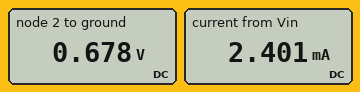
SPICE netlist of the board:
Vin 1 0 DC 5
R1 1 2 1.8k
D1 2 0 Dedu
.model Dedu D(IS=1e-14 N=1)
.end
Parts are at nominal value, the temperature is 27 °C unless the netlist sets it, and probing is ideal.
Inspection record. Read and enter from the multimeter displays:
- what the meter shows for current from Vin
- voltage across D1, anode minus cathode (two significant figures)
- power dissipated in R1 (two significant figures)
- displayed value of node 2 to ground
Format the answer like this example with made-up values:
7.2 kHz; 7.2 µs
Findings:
2.401 mA; 680 mV; 10 mW; 0.678 V
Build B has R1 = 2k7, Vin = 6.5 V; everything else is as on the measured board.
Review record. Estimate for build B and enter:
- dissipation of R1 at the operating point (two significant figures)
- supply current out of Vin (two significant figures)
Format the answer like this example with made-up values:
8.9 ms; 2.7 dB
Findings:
13 mW; 2.2 mA
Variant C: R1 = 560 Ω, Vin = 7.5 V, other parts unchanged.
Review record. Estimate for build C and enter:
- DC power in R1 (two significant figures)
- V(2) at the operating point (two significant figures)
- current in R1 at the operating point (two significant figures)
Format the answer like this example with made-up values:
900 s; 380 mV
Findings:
82 mW; 720 mV; 12 mA
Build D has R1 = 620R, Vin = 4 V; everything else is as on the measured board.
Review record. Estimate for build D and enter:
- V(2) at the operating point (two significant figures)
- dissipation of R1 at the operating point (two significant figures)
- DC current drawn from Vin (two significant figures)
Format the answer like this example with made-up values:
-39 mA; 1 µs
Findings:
700 mV; 18 mW; 5.3 mA
